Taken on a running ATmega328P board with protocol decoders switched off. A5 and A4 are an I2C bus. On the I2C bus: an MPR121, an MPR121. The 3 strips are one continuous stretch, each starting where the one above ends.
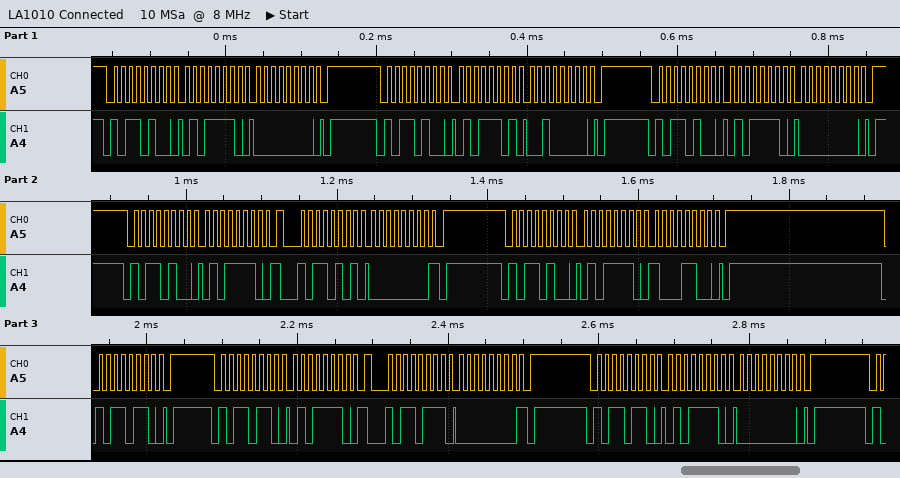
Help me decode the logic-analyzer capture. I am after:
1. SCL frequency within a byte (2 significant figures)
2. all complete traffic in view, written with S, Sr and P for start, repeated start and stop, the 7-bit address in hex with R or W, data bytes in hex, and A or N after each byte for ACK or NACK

100 kHz
S 5AW A 5E A 00 A P S 5AW A 5D A 20 A P S 5AW A 5E A 00 A P S 5AW A 5E A Sr 5AR A 00 N P S 5AW A 5E A 8C A P S 5BW A P S 5BW A 5E A Sr 5BR A 00 N P S 5BW A 5E A 00 A P
